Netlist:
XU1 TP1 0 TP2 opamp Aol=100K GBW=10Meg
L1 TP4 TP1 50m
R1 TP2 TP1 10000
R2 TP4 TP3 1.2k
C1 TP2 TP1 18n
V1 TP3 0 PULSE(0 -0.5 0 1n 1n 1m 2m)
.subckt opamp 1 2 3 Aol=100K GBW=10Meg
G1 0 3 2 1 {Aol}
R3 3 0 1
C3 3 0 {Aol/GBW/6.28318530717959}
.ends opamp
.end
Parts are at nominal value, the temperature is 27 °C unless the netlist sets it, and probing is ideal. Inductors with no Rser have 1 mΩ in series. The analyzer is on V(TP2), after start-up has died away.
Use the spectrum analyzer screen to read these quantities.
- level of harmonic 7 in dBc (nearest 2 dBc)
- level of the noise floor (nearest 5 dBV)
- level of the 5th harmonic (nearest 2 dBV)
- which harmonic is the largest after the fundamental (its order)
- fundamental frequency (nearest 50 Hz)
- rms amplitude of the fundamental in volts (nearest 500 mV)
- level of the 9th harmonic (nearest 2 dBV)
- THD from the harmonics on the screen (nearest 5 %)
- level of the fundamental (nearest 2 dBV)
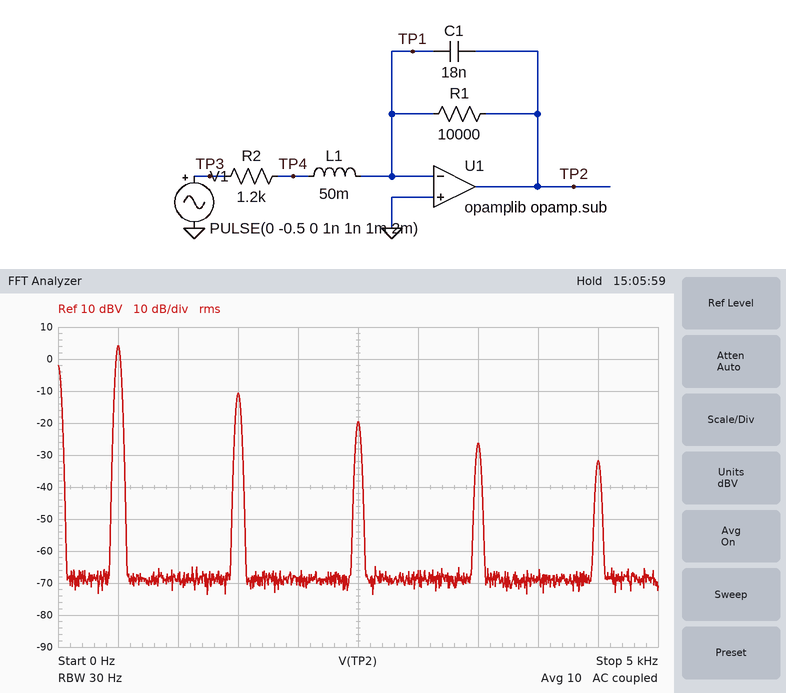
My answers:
-30 dBc
-70 dBV
-20 dBV
3
500 Hz
1.5 V
-32 dBV
20 %
4 dBV
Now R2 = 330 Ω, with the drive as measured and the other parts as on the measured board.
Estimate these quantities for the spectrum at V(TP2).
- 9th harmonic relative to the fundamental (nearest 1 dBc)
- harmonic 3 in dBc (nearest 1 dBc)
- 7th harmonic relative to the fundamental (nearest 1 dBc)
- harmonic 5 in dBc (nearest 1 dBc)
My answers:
-44 dBc
-18 dBc
-38 dBc
-30 dBc
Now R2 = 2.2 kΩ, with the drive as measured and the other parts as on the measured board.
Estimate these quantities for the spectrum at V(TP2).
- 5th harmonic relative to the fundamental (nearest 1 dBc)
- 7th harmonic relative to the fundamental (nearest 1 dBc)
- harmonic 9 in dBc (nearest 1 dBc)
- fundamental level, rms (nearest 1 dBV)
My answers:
-23 dBc
-29 dBc
-34 dBc
-1 dBV
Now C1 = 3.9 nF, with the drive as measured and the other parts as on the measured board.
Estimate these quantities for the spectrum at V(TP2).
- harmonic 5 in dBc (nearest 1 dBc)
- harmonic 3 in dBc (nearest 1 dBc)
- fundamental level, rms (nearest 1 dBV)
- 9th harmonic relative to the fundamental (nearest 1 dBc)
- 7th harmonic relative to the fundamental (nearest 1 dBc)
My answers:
-17 dBc
-11 dBc
5 dBV
-26 dBc
-22 dBc
